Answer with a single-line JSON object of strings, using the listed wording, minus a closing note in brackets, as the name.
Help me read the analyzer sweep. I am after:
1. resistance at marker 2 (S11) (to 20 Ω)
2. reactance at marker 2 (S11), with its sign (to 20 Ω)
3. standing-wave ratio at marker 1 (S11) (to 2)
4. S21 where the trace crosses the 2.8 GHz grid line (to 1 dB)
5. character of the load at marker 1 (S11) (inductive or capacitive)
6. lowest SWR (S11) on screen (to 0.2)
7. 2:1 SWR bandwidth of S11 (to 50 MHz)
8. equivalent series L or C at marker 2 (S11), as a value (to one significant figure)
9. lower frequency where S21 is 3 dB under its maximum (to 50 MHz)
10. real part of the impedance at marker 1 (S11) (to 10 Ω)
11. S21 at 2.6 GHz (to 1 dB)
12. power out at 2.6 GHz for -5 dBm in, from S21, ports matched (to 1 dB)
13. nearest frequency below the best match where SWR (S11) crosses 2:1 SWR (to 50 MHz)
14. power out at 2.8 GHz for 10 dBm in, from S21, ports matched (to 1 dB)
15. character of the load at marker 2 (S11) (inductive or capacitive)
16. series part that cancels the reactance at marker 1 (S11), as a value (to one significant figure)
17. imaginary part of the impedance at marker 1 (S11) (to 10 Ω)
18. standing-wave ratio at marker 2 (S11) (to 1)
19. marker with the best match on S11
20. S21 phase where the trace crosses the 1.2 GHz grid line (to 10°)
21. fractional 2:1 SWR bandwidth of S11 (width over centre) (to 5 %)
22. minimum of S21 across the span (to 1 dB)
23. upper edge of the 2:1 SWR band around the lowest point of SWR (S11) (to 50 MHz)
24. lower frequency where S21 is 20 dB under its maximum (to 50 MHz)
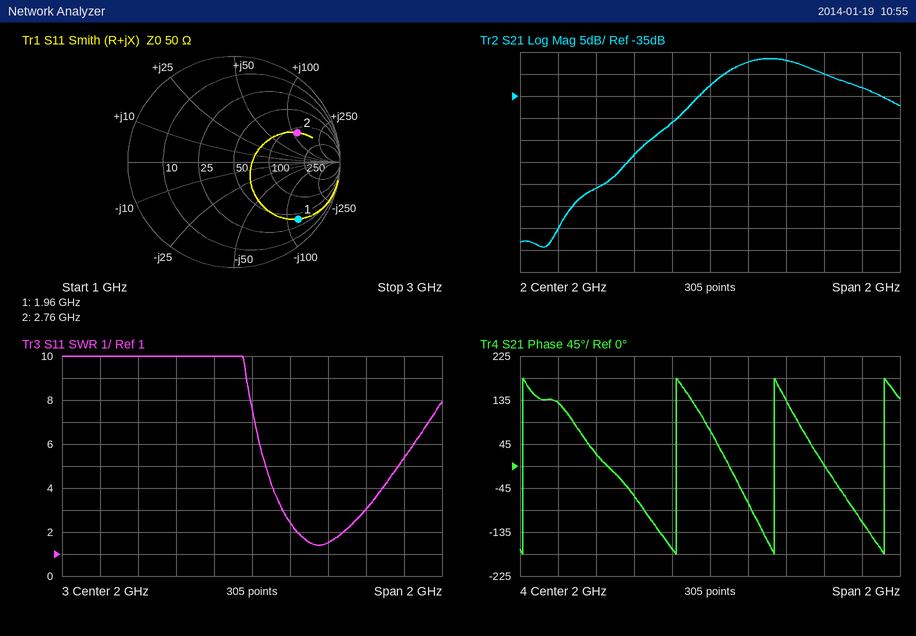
{"resistance at marker 2 (S11)": "120 Ω", "reactance at marker 2 (S11), with its sign": "+120 Ω", "standing-wave ratio at marker 1 (S11)": "10", "S21 where the trace crosses the 2.8 GHz grid line": "-33 dB", "character of the load at marker 1 (S11)": "capacitive", "lowest SWR (S11) on screen": "1.4", "2:1 SWR bandwidth of S11": "250 MHz", "equivalent series L or C at marker 2 (S11), as a value": "7 nH", "lower frequency where S21 is 3 dB under its maximum": "2.10 GHz", "real part of the impedance at marker 1 (S11)": "40 Ω", "S21 at 2.6 GHz": "-30 dB", "power out at 2.6 GHz for -5 dBm in, from S21, ports matched": "-35 dBm", "nearest frequency below the best match where SWR (S11) crosses 2:1 SWR": "2.25 GHz", "power out at 2.8 GHz for 10 dBm in, from S21, ports matched": "-23 dBm", "character of the load at marker 2 (S11)": "inductive", "series part that cancels the reactance at marker 1 (S11), as a value": "10 nH", "imaginary part of the impedance at marker 1 (S11)": "-120 Ω", "standing-wave ratio at marker 2 (S11)": "5", "marker with the best match on S11": "marker 2", "S21 phase where the trace crosses the 1.2 GHz grid line": "130°", "fractional 2:1 SWR bandwidth of S11 (width over centre)": "10 %", "minimum of S21 across the span": "-69 dB", "upper edge of the 2:1 SWR band around the lowest point of SWR (S11)": "2.50 GHz", "lower frequency where S21 is 20 dB under its maximum": "1.65 GHz"}
